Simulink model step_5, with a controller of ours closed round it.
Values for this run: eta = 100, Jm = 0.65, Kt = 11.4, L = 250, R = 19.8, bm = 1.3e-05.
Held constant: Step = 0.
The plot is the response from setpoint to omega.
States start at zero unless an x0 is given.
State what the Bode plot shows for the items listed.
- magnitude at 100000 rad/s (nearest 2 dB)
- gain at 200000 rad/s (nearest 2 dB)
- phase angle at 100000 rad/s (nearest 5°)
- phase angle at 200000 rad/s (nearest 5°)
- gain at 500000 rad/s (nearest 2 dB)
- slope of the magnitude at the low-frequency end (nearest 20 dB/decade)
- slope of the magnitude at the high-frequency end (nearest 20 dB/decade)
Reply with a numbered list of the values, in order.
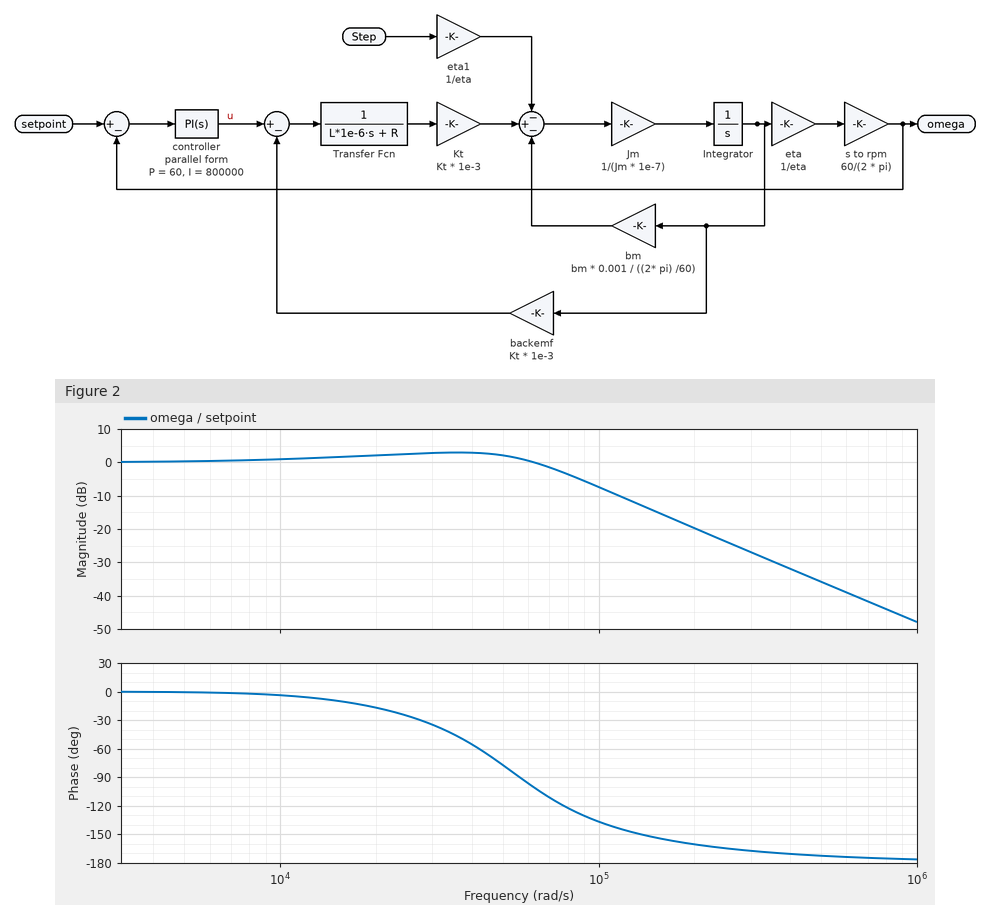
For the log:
1. -8 dB
2. -20 dB
3. -135°
4. -160°
5. -36 dB
6. 0 dB/decade
7. -40 dB/decade
